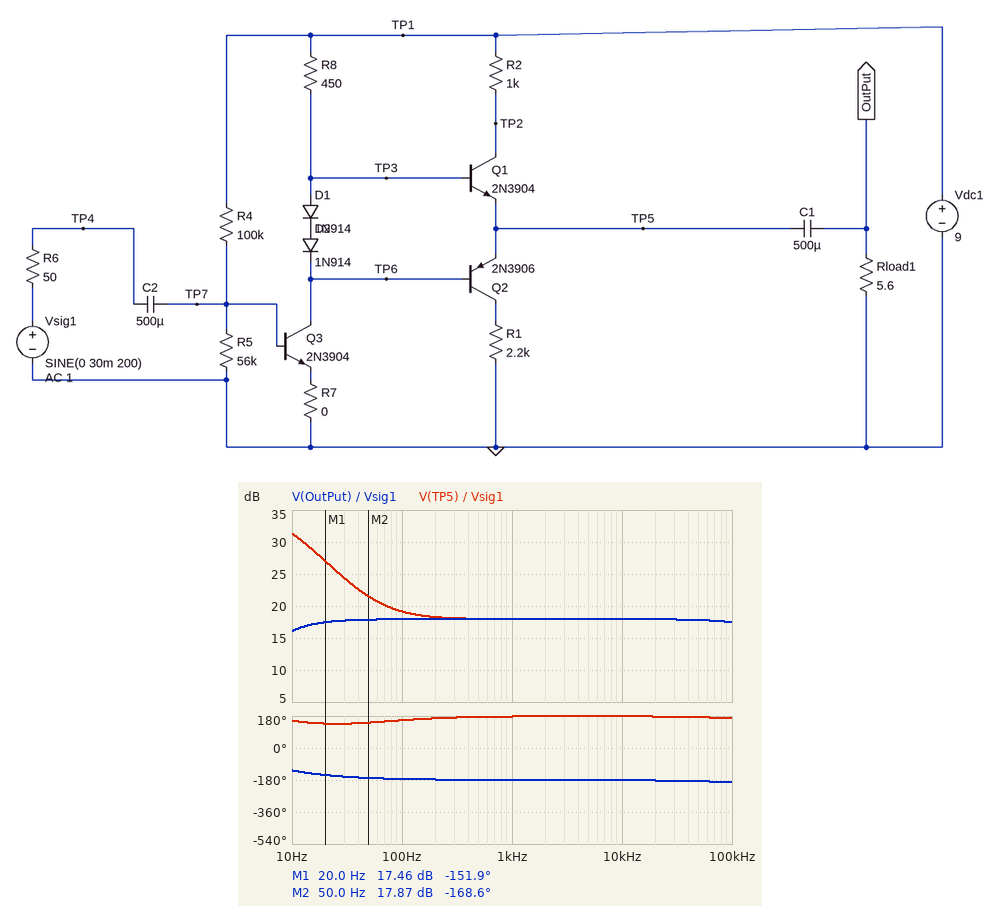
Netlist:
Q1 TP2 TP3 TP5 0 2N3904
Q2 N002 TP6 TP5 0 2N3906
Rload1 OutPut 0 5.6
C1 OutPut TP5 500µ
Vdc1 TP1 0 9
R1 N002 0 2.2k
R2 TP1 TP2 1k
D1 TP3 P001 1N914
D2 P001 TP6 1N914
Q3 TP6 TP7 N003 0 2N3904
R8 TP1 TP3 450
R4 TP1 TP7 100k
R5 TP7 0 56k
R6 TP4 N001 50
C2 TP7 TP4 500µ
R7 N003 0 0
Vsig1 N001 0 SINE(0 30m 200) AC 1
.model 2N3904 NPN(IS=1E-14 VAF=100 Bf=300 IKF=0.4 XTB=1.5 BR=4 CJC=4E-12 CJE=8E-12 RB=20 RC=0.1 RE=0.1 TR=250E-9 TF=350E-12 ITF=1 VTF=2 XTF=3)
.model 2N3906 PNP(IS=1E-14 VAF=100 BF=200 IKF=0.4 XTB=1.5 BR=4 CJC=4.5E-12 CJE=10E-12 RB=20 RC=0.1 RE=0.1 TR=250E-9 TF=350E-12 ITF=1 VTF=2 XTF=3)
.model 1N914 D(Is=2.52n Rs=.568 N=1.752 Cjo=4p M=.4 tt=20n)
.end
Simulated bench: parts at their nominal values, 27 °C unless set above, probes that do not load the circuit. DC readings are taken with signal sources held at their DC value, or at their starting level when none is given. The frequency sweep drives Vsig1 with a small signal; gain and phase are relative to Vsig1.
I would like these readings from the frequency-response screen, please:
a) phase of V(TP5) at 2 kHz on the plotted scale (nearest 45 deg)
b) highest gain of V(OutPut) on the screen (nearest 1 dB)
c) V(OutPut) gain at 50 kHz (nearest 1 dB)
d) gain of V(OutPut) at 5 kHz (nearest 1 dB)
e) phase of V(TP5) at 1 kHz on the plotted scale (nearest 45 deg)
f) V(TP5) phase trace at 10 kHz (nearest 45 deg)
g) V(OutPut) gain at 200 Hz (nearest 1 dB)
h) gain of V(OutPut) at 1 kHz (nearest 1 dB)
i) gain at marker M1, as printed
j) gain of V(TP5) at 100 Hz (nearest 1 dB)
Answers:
180 deg
18 dB
18 dB
18 dB
180 deg
180 deg
18 dB
18 dB
17.46 dB
19 dB
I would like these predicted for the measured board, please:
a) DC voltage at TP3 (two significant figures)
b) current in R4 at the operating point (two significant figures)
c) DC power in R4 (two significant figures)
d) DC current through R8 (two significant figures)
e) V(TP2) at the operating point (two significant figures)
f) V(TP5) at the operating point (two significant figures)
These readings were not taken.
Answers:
1.6 V
83 µA
680 µW
16 mA
6.4 V
950 mV
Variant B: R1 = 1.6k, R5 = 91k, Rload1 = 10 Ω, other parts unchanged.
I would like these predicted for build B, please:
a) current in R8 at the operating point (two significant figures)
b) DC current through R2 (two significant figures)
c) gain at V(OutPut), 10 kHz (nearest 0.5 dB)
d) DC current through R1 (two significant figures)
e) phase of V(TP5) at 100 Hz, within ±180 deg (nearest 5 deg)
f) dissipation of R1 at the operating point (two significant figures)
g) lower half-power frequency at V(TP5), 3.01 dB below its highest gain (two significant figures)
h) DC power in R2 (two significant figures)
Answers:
16 mA
2.7 mA
19.5 dB
570 µA
170 deg
530 µW
2.5 Hz
7.3 mW
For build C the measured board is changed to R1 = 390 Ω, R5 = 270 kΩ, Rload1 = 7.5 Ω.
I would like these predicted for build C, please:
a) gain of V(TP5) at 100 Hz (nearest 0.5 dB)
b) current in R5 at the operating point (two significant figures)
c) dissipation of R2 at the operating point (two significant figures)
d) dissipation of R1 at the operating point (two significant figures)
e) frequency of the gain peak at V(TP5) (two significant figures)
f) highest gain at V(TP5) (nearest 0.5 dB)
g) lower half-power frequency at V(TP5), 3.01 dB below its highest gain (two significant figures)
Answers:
17.5 dB
2.7 µA
16 mW
2.0 mW
8.3 Hz
23.5 dB
2.9 Hz
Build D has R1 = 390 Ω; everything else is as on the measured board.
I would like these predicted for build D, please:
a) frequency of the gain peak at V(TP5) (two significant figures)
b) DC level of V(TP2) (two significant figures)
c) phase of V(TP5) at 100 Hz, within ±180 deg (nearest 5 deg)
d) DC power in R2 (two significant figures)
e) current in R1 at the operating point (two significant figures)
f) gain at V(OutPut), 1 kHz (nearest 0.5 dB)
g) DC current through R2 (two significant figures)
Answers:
6.7 Hz
5.0 V
160 deg
16 mW
2.3 mA
19.0 dB
4.0 mA
